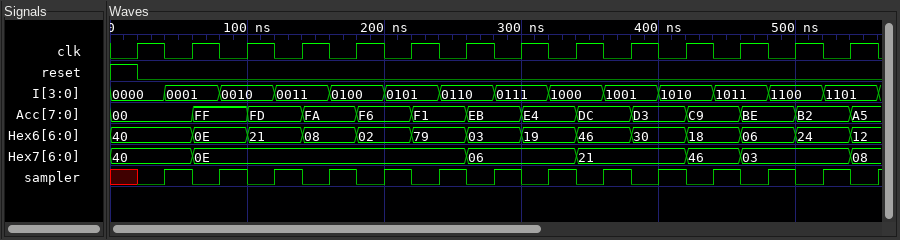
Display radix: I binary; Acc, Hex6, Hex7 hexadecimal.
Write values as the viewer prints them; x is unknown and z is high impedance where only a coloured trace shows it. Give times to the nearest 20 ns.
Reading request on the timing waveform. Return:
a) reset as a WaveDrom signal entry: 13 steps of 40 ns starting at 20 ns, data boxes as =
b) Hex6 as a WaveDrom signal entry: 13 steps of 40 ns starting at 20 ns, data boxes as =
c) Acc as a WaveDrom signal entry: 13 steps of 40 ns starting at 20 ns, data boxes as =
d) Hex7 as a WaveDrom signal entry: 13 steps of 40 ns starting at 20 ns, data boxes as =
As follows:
{name: 'reset', wave: '0............'}
{name: 'Hex6', wave: '=============', data: '40 0E 21 08 02 79 03 19 46 30 18 06 24'}
{name: 'Acc', wave: '=============', data: '00 FF FD FA F6 F1 EB E4 DC D3 C9 BE B2'}
{name: 'Hex7', wave: '==....=.=.==.', data: '40 0E 06 21 46 03'}
